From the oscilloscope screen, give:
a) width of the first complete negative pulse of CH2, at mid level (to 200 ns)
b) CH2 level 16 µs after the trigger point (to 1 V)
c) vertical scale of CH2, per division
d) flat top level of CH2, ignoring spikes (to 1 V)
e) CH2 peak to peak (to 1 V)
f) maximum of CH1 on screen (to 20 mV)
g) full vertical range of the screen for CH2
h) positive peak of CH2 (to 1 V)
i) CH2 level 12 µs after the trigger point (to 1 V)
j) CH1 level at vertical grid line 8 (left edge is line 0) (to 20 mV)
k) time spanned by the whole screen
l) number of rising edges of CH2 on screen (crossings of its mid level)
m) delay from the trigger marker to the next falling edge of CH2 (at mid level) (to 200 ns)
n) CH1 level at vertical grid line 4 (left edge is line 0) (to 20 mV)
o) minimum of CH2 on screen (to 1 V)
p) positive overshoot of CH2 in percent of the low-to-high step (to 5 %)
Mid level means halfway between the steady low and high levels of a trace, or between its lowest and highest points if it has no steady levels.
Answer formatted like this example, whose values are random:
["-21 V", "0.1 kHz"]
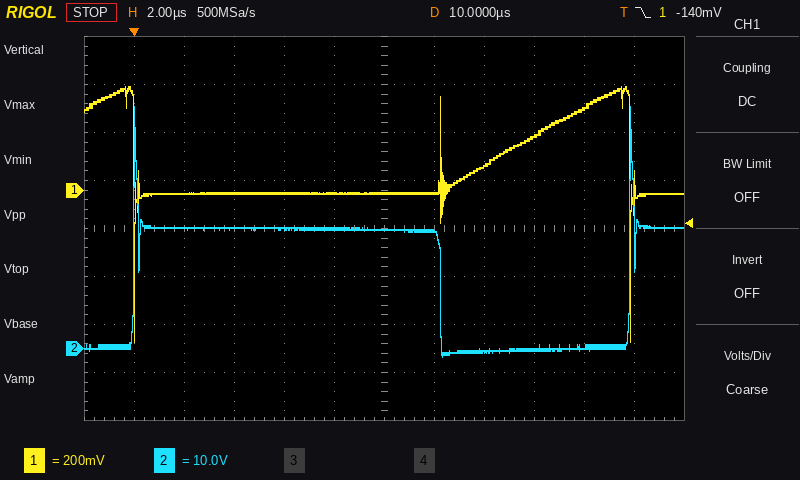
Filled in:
["7.6 µs", "0 V", "10 V", "25 V", "52 V", "440 mV", "80 V", "50 V", "24 V", "100 mV", "24 µs", "2", "12.2 µs", "-20 mV", "-2 V", "100 %"]
